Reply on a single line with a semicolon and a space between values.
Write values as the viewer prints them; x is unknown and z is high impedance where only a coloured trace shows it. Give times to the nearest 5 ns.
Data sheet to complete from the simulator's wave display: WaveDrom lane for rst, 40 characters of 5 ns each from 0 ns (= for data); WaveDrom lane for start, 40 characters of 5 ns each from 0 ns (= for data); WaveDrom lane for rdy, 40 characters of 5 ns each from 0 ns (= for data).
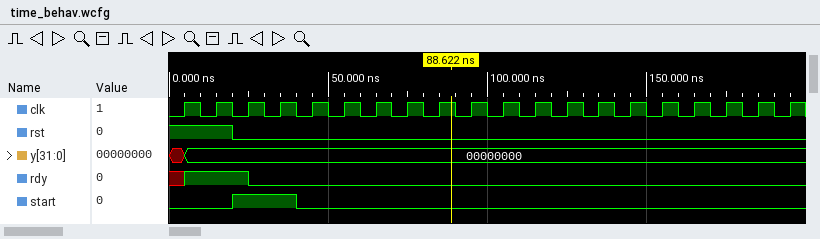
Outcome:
{name: 'rst', wave: '1...0...................................'}; {name: 'start', wave: '0...1...0...............................'}; {name: 'rdy', wave: 'x1...0..................................'}
